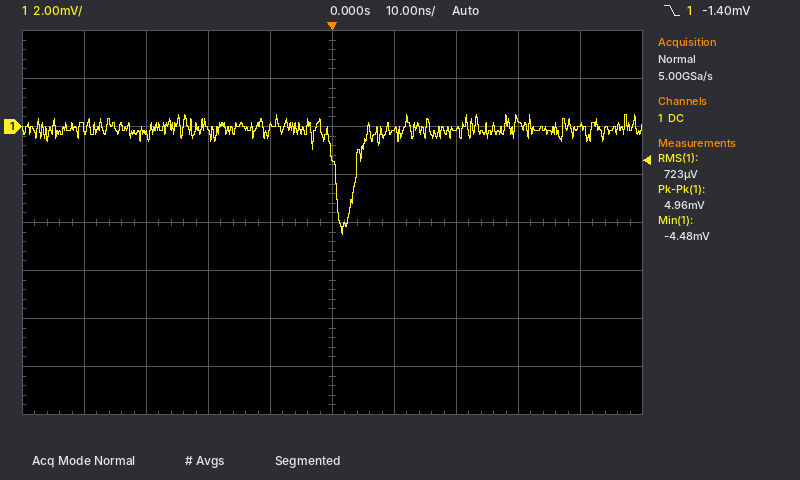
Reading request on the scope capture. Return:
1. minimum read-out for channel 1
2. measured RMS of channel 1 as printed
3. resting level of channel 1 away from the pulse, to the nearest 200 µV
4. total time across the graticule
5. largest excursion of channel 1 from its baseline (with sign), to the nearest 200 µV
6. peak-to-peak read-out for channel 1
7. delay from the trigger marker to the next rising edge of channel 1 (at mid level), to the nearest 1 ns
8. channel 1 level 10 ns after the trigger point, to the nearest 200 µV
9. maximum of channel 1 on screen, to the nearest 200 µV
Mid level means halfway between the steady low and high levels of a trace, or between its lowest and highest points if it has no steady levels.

-4.48 mV
723 µV
-200 µV
100 ns
-4.4 mV
4.96 mV
4 ns
-200 µV
400 µV
